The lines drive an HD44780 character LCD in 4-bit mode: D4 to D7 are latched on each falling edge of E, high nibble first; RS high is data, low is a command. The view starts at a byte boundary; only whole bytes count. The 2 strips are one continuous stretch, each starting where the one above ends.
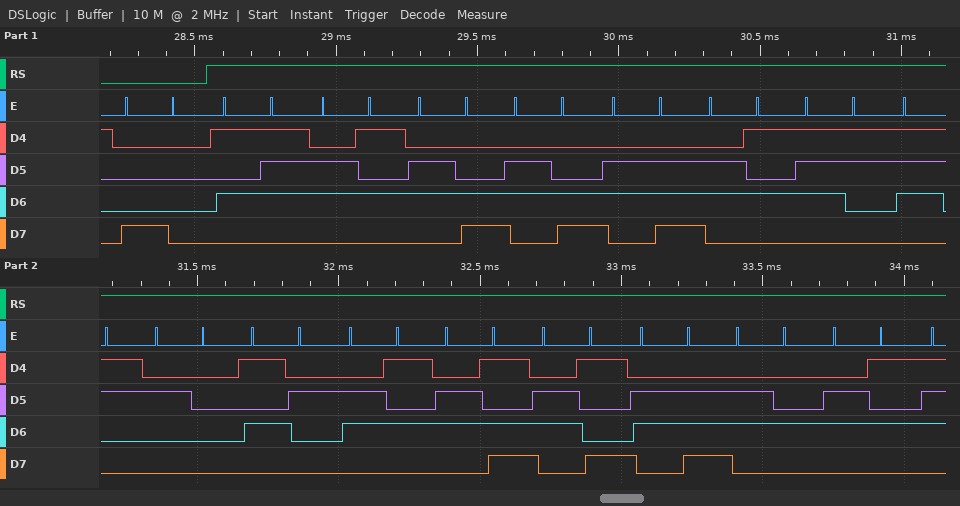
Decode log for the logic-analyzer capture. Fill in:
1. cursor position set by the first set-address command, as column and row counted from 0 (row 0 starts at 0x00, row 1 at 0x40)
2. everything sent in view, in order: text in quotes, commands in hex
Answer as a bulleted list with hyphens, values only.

- column 0, row 0
- 0x80 "Wellness Reminde"
